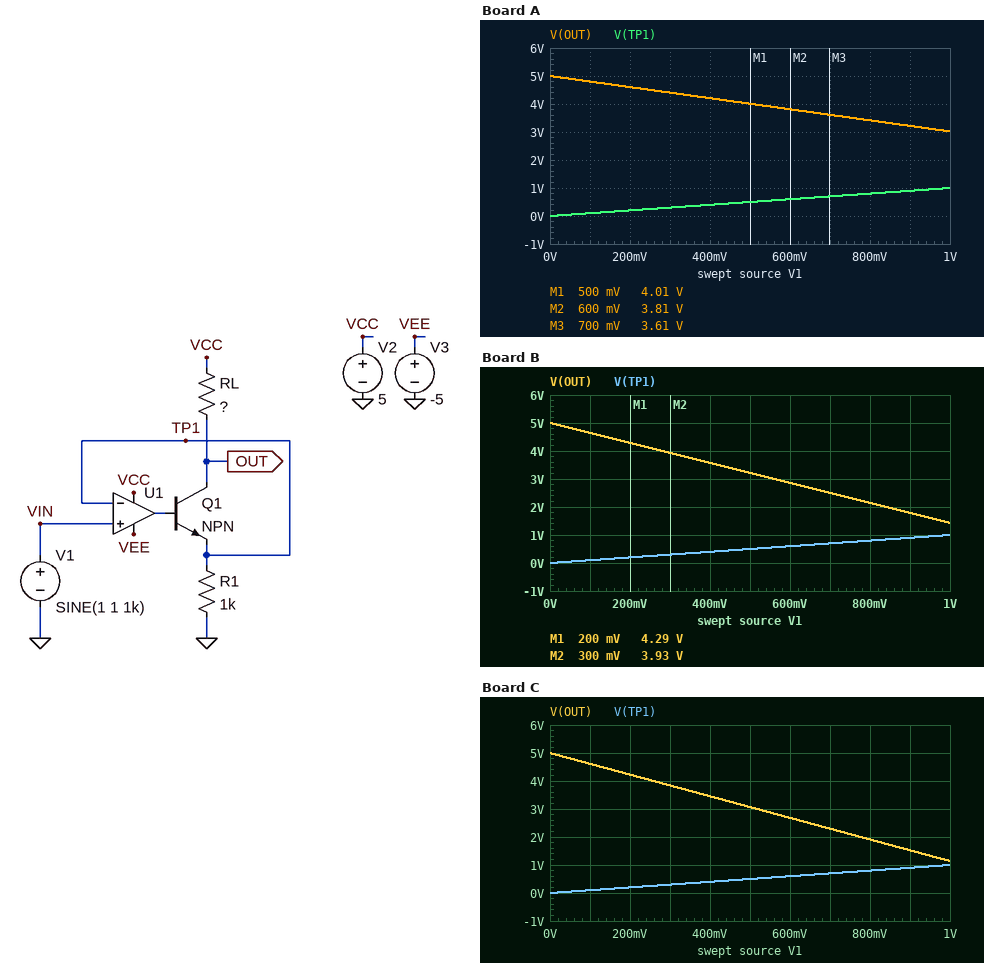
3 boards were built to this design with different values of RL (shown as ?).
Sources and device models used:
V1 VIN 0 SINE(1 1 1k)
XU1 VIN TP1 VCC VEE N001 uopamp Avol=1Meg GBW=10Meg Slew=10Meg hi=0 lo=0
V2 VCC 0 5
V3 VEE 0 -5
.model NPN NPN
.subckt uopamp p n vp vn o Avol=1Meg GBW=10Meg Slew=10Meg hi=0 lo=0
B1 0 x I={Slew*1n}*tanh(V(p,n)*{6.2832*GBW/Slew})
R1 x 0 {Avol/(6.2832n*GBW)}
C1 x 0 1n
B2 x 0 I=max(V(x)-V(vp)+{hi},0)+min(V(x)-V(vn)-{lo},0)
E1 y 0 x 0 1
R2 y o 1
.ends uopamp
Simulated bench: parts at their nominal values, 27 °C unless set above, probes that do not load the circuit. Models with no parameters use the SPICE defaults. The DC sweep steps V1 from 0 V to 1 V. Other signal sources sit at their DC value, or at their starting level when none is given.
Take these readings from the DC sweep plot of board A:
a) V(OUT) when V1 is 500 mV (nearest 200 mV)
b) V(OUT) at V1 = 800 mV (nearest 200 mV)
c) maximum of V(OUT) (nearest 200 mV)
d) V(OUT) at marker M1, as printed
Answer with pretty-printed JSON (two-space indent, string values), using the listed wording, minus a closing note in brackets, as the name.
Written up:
{
  "V(OUT) when V1 is 500 mV": "4.0 V",
  "V(OUT) at V1 = 800 mV": "3.4 V",
  "maximum of V(OUT)": "5.0 V",
  "V(OUT) at marker M1, as printed": "4.01 V"
}
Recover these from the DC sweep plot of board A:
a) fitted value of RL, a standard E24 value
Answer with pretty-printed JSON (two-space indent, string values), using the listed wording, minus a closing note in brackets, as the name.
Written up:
{
  "fitted value of RL, a standard E24 value": "2 kΩ"
}
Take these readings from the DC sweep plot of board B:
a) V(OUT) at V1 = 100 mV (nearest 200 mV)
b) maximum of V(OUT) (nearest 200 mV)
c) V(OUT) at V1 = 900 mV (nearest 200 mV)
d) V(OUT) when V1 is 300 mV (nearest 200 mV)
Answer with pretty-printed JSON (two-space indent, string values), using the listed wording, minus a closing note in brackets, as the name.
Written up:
{
  "V(OUT) at V1 = 100 mV": "4.6 V",
  "maximum of V(OUT)": "5.0 V",
  "V(OUT) at V1 = 900 mV": "1.8 V",
  "V(OUT) when V1 is 300 mV": "4.0 V"
}
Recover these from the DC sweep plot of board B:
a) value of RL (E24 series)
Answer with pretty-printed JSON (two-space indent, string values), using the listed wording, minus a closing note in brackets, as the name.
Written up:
{
  "value of RL": "3.6 kΩ"
}
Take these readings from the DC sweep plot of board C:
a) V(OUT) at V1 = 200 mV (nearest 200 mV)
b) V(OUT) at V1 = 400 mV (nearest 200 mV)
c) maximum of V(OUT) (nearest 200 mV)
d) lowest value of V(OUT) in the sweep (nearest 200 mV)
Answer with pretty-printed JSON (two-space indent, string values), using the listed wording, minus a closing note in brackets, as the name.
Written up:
{
  "V(OUT) at V1 = 200 mV": "4.2 V",
  "V(OUT) at V1 = 400 mV": "3.4 V",
  "maximum of V(OUT)": "5.0 V",
  "lowest value of V(OUT) in the sweep": "1.2 V"
}
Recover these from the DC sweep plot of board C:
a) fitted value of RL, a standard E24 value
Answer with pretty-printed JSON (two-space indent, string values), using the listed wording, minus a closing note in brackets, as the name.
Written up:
{
  "fitted value of RL, a standard E24 value": "3.9 kΩ"
}
